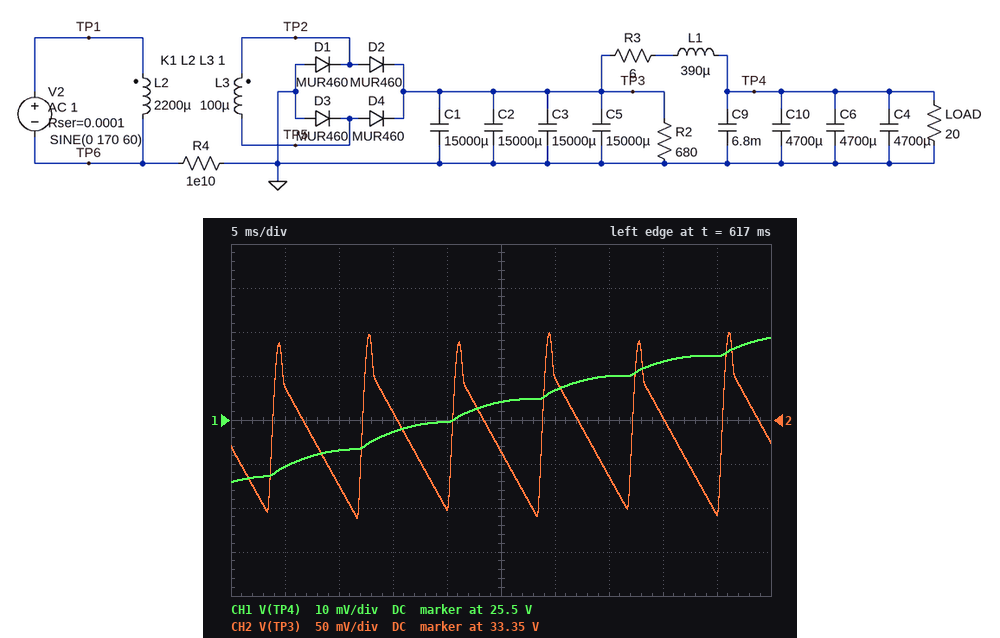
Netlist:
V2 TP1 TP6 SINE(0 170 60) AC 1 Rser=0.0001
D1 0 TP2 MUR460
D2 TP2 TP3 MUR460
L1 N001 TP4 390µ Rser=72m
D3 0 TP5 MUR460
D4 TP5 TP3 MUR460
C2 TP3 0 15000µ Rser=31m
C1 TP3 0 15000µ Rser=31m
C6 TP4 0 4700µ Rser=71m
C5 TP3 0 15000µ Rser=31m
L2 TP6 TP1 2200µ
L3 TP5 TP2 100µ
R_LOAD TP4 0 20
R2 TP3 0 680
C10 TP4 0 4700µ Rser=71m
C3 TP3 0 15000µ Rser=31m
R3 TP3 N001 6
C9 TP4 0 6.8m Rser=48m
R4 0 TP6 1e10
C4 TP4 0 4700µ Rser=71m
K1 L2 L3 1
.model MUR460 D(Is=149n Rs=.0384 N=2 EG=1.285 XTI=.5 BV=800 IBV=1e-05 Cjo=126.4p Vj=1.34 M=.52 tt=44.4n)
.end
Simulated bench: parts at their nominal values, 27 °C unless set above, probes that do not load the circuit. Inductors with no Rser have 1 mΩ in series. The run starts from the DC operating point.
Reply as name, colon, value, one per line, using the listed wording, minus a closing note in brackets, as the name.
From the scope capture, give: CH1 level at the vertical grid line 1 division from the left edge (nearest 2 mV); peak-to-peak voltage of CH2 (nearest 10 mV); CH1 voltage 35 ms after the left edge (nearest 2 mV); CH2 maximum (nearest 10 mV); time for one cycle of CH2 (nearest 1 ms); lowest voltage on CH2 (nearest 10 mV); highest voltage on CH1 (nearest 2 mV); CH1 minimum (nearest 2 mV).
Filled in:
CH1 level at the vertical grid line 1 division from the left edge: 25.490 V
peak-to-peak voltage of CH2: 210 mV
CH1 voltage 35 ms after the left edge: 25.510 V
CH2 maximum: 33.45 V
time for one cycle of CH2: 8 ms
lowest voltage on CH2: 33.24 V
highest voltage on CH1: 25.518 V
CH1 minimum: 25.486 V
